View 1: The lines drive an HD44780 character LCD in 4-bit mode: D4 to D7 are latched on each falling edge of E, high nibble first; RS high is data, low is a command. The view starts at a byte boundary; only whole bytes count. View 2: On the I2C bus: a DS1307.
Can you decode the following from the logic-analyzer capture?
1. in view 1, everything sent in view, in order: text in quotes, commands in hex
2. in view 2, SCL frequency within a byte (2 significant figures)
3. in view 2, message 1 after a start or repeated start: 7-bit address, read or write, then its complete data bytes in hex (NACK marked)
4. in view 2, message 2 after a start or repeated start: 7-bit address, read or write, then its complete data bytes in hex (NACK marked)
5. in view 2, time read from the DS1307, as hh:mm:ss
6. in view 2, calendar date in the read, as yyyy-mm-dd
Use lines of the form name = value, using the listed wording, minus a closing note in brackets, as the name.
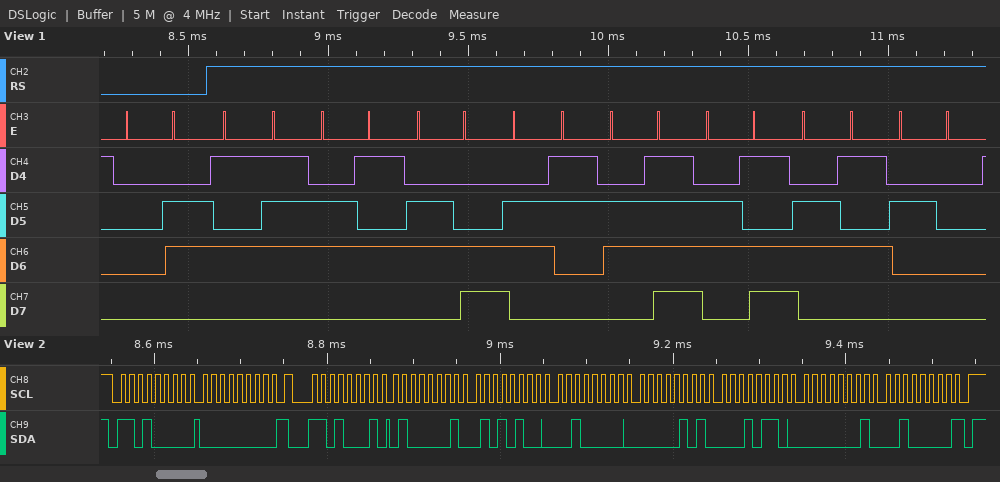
in view 1, everything sent in view, in order: text in quotes, commands in hex = 0x06 "Welcome "
in view 2, SCL frequency within a byte = 100 kHz
in view 2, message 1 after a start or repeated start: 7-bit address, read or write, then its complete data bytes in hex = 0x68 write: 00
in view 2, message 2 after a start or repeated start: 7-bit address, read or write, then its complete data bytes in hex = 0x68 read: 41 54 20 05 16 01 20 NACK
in view 2, time read from the DS1307, as hh:mm:ss = 20:54:41
in view 2, calendar date in the read, as yyyy-mm-dd = 2020-01-16
